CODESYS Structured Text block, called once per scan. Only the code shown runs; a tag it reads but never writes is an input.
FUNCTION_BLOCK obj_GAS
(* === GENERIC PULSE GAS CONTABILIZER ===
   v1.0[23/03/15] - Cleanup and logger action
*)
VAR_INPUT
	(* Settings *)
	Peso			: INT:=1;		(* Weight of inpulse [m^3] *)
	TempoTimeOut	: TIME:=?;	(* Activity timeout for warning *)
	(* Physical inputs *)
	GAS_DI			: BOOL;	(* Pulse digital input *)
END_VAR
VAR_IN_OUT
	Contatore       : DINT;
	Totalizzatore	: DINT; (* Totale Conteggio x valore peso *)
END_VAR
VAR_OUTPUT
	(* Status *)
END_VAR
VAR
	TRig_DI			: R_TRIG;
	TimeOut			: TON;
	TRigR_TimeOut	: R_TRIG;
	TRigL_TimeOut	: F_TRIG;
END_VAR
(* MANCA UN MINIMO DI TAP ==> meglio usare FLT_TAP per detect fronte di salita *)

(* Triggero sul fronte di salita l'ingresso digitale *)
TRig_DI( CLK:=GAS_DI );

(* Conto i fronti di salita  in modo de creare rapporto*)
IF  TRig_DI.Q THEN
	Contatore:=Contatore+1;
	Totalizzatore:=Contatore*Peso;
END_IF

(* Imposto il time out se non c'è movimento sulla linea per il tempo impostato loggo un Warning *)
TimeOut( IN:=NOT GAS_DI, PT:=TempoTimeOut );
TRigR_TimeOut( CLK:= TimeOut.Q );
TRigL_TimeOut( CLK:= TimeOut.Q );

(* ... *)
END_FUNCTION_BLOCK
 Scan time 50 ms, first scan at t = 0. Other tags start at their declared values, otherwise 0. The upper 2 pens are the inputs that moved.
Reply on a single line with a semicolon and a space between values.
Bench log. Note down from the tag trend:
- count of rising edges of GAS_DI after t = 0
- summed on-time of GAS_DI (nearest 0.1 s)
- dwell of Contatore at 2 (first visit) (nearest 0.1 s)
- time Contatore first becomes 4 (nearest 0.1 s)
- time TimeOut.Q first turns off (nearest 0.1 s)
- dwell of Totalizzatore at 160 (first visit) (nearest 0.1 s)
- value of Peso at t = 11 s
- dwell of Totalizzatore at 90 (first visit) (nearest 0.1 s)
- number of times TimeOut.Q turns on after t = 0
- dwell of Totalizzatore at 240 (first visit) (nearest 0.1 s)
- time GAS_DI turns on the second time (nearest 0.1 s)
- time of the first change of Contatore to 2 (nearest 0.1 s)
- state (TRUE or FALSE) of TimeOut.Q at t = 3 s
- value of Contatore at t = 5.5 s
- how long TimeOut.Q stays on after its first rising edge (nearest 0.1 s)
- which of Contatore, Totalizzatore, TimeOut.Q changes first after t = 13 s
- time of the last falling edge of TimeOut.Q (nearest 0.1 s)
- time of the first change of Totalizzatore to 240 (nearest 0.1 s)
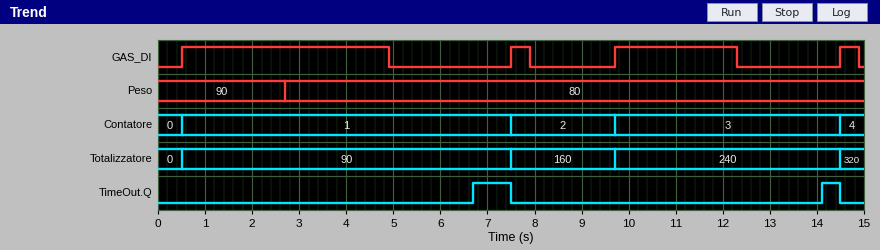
4; 7.8 s; 2.2 s; 14.5 s; 7.5 s; 2.2 s; 80; 7.0 s; 2; 4.8 s; 7.5 s; 7.5 s; FALSE; 1; 0.8 s; TimeOut.Q; 14.5 s; 9.7 s
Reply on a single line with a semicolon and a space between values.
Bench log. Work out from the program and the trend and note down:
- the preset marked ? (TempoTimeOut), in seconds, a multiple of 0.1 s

1.8 s
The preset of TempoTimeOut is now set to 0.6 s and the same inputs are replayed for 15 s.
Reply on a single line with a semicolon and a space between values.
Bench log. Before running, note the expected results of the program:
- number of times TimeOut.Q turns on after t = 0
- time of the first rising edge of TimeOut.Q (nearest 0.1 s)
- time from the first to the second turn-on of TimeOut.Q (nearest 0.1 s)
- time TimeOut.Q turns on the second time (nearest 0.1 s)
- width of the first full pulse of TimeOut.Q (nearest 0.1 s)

3; 5.5 s; 3.0 s; 8.5 s; 2.0 s
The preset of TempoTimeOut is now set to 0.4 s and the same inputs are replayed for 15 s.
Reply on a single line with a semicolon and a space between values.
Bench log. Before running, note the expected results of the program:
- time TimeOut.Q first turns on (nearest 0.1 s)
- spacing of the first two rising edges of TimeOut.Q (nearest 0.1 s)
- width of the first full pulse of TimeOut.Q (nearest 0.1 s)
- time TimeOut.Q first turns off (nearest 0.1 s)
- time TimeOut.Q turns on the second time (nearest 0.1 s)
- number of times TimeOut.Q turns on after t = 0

0.4 s; 4.9 s; 0.1 s; 0.5 s; 5.3 s; 4
